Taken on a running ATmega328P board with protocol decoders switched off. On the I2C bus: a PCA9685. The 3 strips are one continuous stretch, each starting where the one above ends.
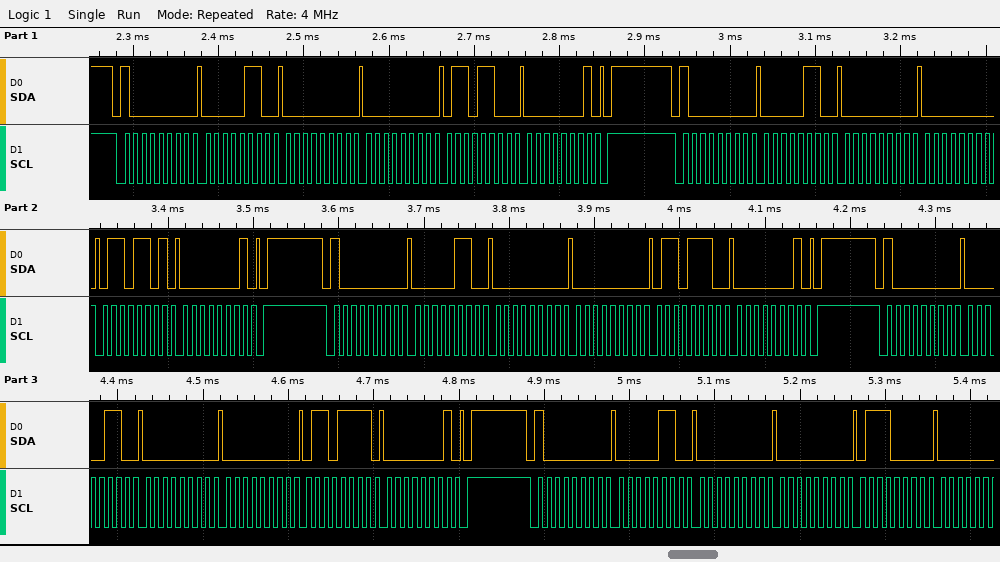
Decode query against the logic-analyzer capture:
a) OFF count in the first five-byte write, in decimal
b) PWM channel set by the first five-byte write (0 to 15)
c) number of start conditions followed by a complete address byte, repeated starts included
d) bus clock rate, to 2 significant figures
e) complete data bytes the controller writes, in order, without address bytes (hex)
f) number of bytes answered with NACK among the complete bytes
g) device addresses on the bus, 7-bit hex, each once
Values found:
364
0
5
100 kHz
06 00 00 6C 01 06 00 00 6D 01 06 00 00 6E 01 06 00 00 6F 01 06 00 00 70
0
0x40
